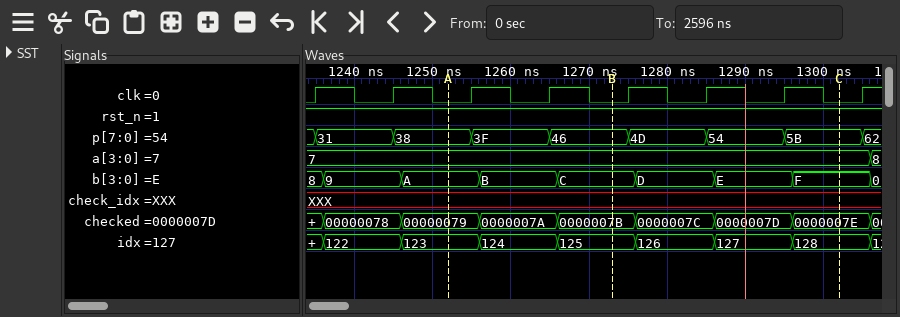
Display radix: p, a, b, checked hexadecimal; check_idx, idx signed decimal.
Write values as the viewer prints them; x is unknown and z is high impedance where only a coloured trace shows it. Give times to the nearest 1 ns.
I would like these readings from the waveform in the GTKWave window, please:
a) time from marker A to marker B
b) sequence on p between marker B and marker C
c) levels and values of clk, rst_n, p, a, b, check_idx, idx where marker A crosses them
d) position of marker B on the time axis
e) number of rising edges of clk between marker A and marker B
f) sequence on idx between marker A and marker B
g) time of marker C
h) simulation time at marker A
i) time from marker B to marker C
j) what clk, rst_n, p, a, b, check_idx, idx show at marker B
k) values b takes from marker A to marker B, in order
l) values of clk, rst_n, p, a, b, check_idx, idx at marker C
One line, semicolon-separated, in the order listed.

21 ns; 46, 4D, 54, 5B; clk=0, rst_n=1, p=38, a=7, b=A, check_idx=XXX, idx=123; 1273 ns; 2; 123, 124, 125; 1302 ns; 1252 ns; 29 ns; clk=0, rst_n=1, p=46, a=7, b=C, check_idx=XXX, idx=125; A, B, C; clk=0, rst_n=1, p=5B, a=7, b=F, check_idx=XXX, idx=128
